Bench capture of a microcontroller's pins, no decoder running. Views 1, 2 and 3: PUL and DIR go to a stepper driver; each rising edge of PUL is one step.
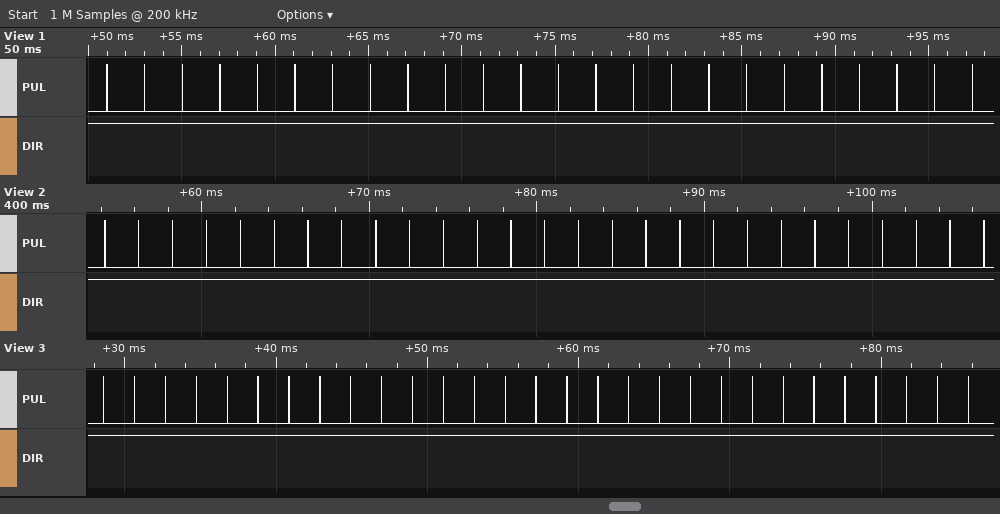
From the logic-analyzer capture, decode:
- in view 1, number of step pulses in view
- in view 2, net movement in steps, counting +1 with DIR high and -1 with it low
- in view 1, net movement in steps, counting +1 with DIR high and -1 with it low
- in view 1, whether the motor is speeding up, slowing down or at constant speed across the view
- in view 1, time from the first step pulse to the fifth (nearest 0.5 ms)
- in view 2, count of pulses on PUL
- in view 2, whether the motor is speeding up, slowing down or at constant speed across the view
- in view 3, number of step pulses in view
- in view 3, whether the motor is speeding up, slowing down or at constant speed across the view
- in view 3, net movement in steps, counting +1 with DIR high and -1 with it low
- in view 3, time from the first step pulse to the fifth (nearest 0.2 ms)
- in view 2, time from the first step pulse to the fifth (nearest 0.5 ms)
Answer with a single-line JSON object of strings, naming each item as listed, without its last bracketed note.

{"in view 1, number of step pulses in view": "24", "in view 2, net movement in steps, counting +1 with DIR high and -1 with it low": "+27", "in view 1, net movement in steps, counting +1 with DIR high and -1 with it low": "+24", "in view 1, whether the motor is speeding up, slowing down or at constant speed across the view": "constant speed", "in view 1, time from the first step pulse to the fifth": "8.0 ms", "in view 2, count of pulses on PUL": "27", "in view 2, whether the motor is speeding up, slowing down or at constant speed across the view": "constant speed", "in view 3, number of step pulses in view": "29", "in view 3, whether the motor is speeding up, slowing down or at constant speed across the view": "constant speed", "in view 3, net movement in steps, counting +1 with DIR high and -1 with it low": "+29", "in view 3, time from the first step pulse to the fifth": "8.2 ms", "in view 2, time from the first step pulse to the fifth": "8.0 ms"}
